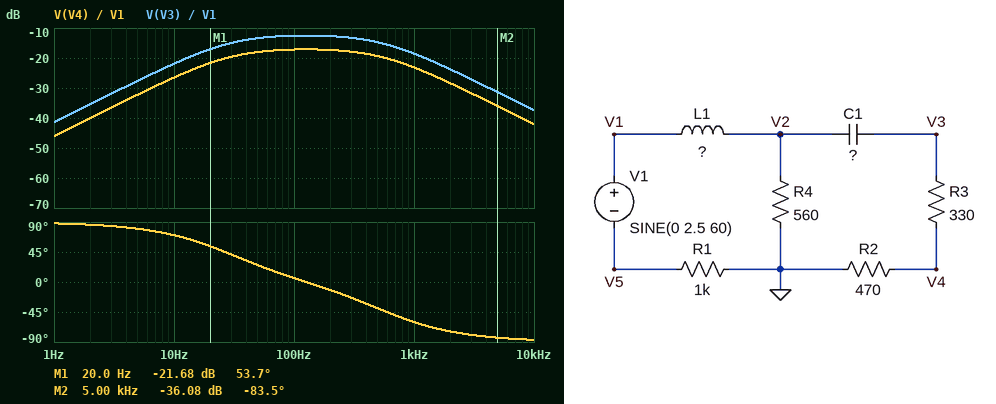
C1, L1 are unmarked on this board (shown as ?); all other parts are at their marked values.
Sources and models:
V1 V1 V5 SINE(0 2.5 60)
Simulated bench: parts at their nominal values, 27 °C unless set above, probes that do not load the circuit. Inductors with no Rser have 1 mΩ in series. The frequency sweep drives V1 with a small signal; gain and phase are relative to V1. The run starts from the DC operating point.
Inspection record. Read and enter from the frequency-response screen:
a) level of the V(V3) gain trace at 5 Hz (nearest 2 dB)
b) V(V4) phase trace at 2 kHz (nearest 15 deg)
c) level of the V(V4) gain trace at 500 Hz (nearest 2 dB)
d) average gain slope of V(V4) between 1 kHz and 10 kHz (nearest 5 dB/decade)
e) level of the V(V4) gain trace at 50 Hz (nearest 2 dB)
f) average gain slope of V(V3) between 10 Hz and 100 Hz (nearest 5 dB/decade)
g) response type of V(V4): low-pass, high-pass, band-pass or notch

-28 dB
-75 deg
-20 dB
-20 dB/decade
-18 dB
10 dB/decade
band-pass
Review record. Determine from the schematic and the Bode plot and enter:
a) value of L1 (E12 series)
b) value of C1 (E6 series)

390 mH
4.7 µF
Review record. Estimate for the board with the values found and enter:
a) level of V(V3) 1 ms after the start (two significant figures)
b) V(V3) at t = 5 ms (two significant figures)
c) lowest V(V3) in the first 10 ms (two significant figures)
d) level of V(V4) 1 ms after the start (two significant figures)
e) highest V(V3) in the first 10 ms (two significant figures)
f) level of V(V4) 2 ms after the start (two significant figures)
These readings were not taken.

150 mV
340 mV
-500 mV
90 mV
420 mV
190 mV
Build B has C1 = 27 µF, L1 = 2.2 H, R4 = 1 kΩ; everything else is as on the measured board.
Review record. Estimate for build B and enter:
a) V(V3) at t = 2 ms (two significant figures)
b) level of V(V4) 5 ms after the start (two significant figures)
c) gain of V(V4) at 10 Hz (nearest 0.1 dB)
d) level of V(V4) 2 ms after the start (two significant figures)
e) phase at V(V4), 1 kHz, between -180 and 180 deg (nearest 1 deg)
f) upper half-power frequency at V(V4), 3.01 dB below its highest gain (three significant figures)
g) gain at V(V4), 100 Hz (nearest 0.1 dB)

240 mV
370 mV
-15.6 dB
140 mV
-84 deg
112 Hz
-17.6 dB
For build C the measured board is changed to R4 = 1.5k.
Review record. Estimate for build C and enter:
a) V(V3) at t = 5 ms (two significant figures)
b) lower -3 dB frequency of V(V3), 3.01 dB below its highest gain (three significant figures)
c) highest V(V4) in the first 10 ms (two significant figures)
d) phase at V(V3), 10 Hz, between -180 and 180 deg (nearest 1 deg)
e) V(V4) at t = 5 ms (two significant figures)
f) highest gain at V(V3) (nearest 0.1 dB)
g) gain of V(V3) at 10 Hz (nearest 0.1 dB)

510 mV
22.8 Hz
360 mV
67 deg
300 mV
-9.5 dB
-17.6 dB
